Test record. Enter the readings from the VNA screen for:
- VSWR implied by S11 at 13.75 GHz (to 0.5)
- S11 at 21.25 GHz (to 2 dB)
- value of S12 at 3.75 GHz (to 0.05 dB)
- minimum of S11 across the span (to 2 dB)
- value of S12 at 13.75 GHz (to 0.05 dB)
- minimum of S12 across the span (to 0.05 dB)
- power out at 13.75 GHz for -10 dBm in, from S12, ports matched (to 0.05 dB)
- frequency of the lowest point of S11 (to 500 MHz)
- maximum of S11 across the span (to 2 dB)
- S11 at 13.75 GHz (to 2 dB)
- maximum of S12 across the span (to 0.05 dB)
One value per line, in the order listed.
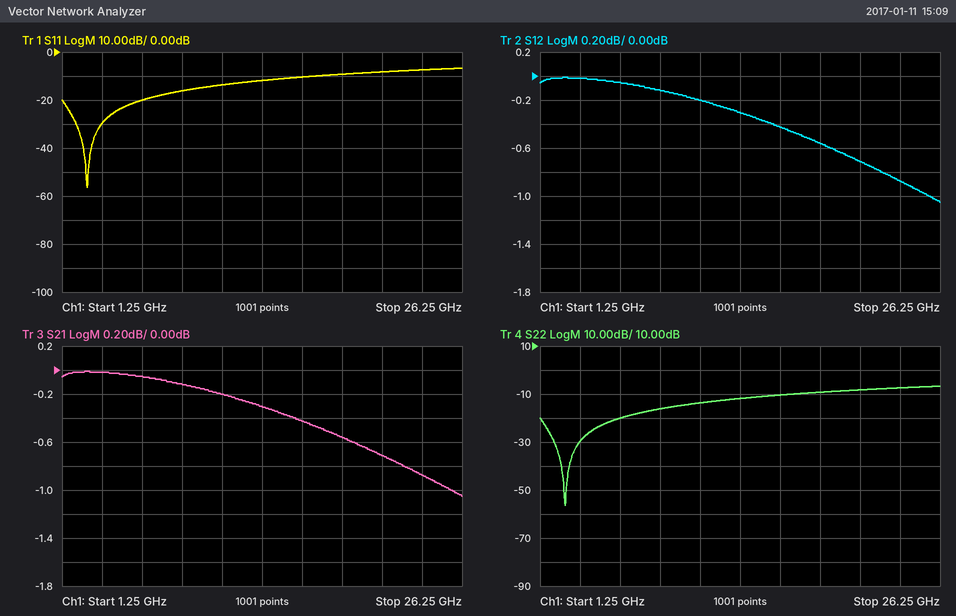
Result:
1.5
-8 dB
0.00 dB
-56 dB
-0.30 dB
-1.05 dB
-10.30 dBm
3.0 GHz
-6 dB
-12 dB
0.00 dB
